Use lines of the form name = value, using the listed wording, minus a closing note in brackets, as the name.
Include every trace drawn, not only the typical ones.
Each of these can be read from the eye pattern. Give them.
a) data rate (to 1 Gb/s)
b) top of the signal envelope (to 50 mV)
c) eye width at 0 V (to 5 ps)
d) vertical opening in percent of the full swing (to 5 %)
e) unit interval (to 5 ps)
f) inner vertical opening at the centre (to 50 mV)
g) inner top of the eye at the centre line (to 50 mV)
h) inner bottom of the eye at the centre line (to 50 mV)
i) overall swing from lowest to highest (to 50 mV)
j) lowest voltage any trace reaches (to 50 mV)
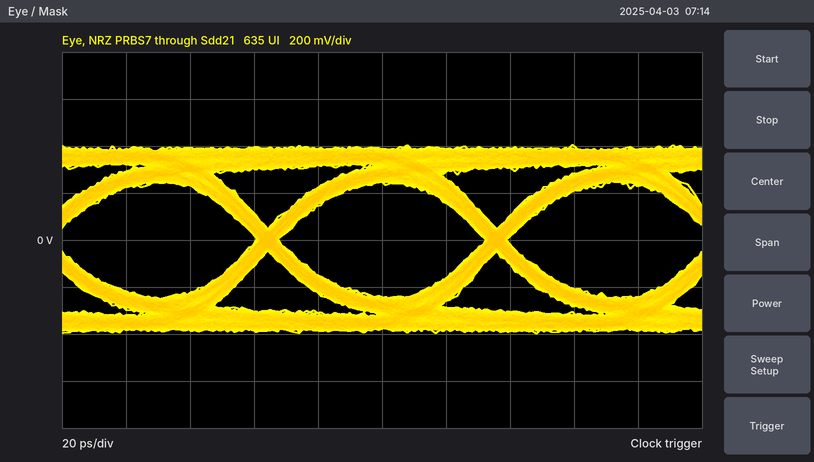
data rate = 14 Gb/s
top of the signal envelope = 400 mV
eye width at 0 V = 65 ps
vertical opening in percent of the full swing = 60 %
unit interval = 70 ps
inner vertical opening at the centre = 500 mV
inner top of the eye at the centre line = 250 mV
inner bottom of the eye at the centre line = -250 mV
overall swing from lowest to highest = 800 mV
lowest voltage any trace reaches = -400 mV
